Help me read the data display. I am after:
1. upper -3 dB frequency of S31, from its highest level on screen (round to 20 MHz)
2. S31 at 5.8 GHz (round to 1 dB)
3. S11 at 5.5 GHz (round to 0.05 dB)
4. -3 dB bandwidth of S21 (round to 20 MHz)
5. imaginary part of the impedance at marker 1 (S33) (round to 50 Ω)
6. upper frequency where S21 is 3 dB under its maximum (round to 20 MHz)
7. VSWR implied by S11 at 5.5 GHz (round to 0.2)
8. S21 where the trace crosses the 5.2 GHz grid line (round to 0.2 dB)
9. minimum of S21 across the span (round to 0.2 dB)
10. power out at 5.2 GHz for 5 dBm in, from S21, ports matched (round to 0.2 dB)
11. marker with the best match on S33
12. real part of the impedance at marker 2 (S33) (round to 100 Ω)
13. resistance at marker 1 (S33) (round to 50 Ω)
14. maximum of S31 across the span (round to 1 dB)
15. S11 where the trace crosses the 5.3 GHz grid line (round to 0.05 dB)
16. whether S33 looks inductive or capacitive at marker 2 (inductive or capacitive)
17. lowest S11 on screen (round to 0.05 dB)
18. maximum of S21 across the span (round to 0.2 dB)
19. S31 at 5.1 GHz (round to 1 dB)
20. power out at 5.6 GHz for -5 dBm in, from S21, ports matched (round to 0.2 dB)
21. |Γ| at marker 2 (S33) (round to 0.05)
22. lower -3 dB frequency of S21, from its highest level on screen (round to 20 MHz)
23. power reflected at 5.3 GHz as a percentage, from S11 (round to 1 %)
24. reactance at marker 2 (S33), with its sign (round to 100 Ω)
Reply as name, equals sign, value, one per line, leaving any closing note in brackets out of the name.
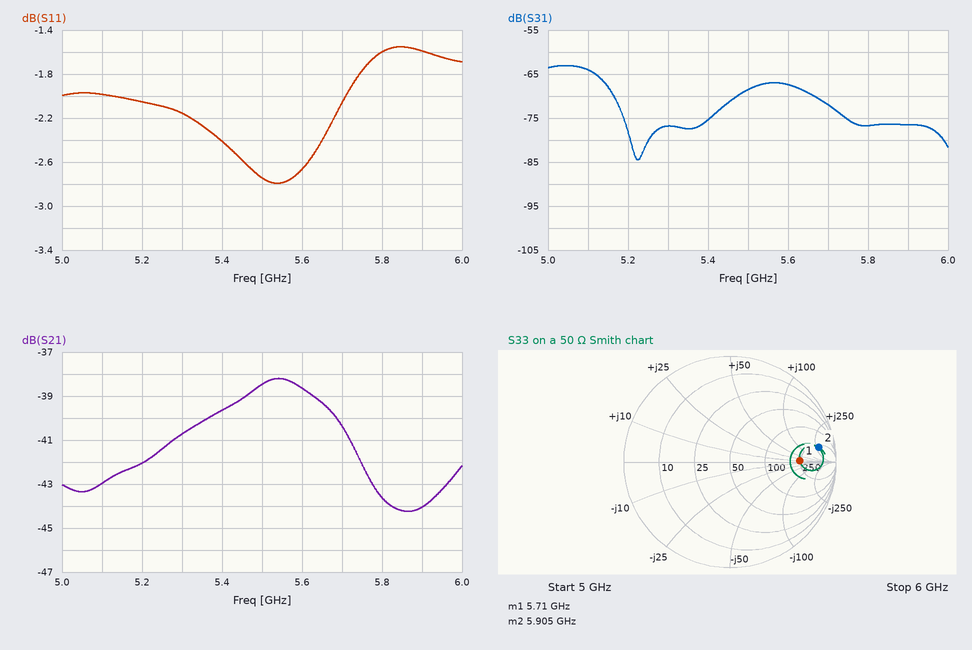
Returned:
upper -3 dB frequency of S31, from its highest level on screen = 5.14 GHz
S31 at 5.8 GHz = -77 dB
S11 at 5.5 GHz = -2.75 dB
-3 dB bandwidth of S21 = 460 MHz
imaginary part of the impedance at marker 1 (S33) = 0 Ω
upper frequency where S21 is 3 dB under its maximum = 5.72 GHz
VSWR implied by S11 at 5.5 GHz = 6.4
S21 where the trace crosses the 5.2 GHz grid line = -42.0 dB
minimum of S21 across the span = -44.2 dB
power out at 5.2 GHz for 5 dBm in, from S21, ports matched = -37.0 dBm
marker with the best match on S33 = marker 1
real part of the impedance at marker 2 (S33) = 300 Ω
resistance at marker 1 (S33) = 250 Ω
maximum of S31 across the span = -63 dB
S11 where the trace crosses the 5.3 GHz grid line = -2.15 dB
whether S33 looks inductive or capacitive at marker 2 = inductive
lowest S11 on screen = -2.80 dB
maximum of S21 across the span = -38.2 dB
S31 at 5.1 GHz = -64 dB
power out at 5.6 GHz for -5 dBm in, from S21, ports matched = -43.6 dBm
|Γ| at marker 2 (S33) = 0.85
lower -3 dB frequency of S21, from its highest level on screen = 5.26 GHz
power reflected at 5.3 GHz as a percentage, from S11 = 61 %
reactance at marker 2 (S33), with its sign = +300 Ω
